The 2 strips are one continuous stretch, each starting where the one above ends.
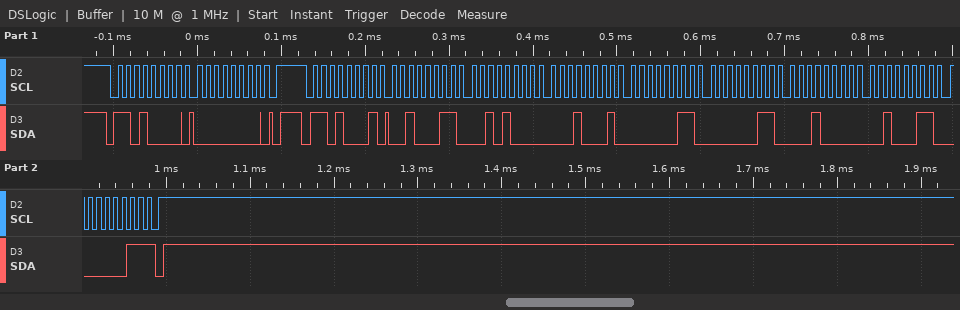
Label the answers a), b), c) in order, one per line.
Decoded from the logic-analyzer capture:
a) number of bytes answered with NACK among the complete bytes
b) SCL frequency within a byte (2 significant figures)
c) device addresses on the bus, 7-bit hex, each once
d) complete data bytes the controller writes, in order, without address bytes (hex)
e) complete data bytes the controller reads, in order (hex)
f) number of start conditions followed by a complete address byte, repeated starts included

a) 1
b) 100 kHz
c) 0x68
d) 00
e) 23 28 11 03 03 10 23 03
f) 2
